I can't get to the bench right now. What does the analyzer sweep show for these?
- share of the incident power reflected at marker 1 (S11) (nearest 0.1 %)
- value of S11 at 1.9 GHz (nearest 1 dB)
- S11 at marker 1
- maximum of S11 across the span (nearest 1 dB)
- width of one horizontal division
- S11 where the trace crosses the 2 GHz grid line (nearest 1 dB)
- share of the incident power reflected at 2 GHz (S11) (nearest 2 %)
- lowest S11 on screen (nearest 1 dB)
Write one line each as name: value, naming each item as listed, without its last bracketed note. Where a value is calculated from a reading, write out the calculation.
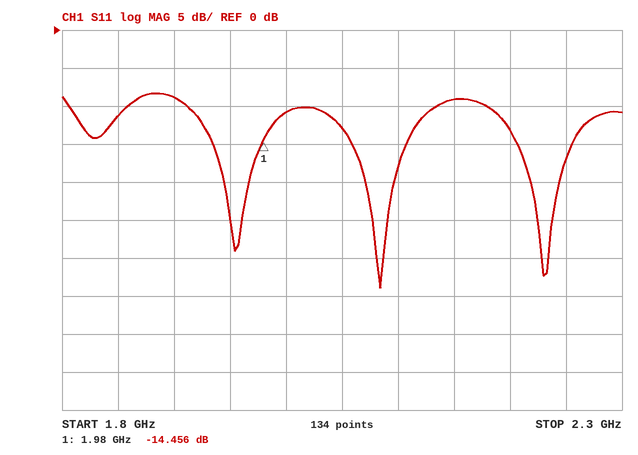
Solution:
share of the incident power reflected at marker 1 (S11): 10^(-14.456/10) ≈ 3.6 %
value of S11 at 1.9 GHz: -9 dB
S11 at marker 1: -14.456 dB
maximum of S11 across the span: -8 dB
width of one horizontal division: 50 MHz
S11 where the trace crosses the 2 GHz grid line: -11 dB
share of the incident power reflected at 2 GHz (S11): 10^(-11/10) ≈ 8 %
lowest S11 on screen: -34 dB
